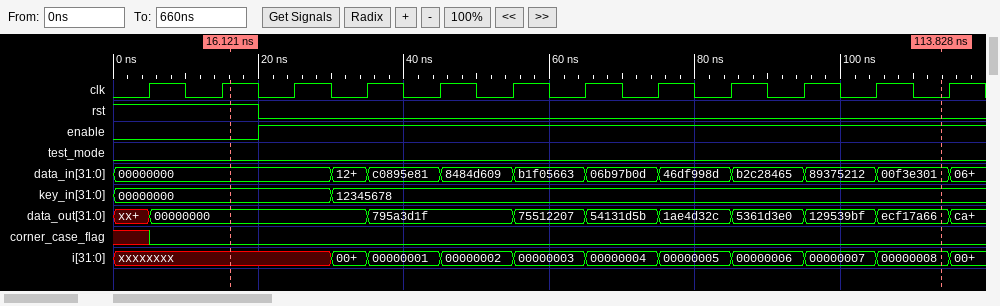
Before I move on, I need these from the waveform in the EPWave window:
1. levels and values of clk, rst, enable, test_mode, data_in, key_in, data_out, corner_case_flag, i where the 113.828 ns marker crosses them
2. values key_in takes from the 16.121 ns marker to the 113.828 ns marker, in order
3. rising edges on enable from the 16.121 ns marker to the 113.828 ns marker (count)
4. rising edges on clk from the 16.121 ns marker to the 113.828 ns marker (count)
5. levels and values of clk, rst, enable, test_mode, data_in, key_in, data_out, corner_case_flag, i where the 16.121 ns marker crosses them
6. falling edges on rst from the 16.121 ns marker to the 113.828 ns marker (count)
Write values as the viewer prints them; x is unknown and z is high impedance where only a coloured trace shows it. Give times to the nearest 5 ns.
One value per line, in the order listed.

clk=0, rst=0, enable=1, test_mode=0, data_in=00f3e301, key_in=12345678, data_out=ecf17a66, corner_case_flag=0, i=00000008
00000000, 12345678
1
9
clk=1, rst=1, enable=0, test_mode=0, data_in=00000000, key_in=00000000, data_out=00000000, corner_case_flag=0, i=xxxxxxxx
1
